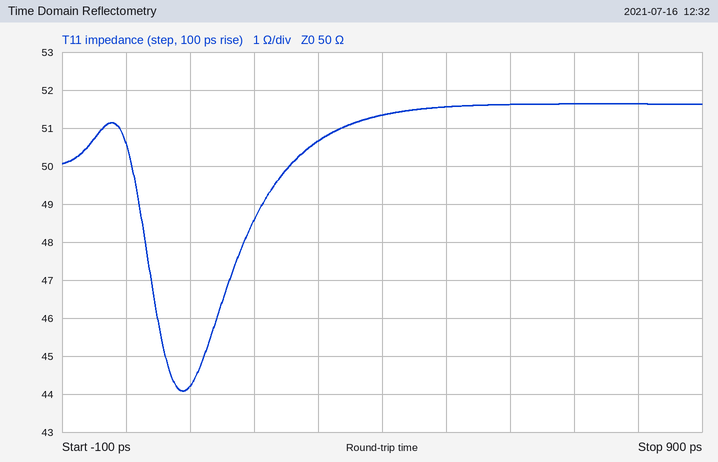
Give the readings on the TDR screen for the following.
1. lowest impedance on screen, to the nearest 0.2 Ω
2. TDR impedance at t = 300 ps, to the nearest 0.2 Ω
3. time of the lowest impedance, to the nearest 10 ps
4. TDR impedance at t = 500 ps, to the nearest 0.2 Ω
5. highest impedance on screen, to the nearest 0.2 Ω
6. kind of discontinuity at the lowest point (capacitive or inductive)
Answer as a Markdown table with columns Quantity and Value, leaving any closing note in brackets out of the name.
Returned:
| Quantity | Value |
|---|---|
| lowest impedance on screen, to the nearest 0.2 Ω | 44.0 Ω |
| TDR impedance at t = 300 ps, to the nearest 0.2 Ω | 50.6 Ω |
| time of the lowest impedance, to the nearest 10 ps | 90 ps |
| TDR impedance at t = 500 ps, to the nearest 0.2 Ω | 51.6 Ω |
| highest impedance on screen, to the nearest 0.2 Ω | 51.6 Ω |
| kind of discontinuity at the lowest point | capacitive |
